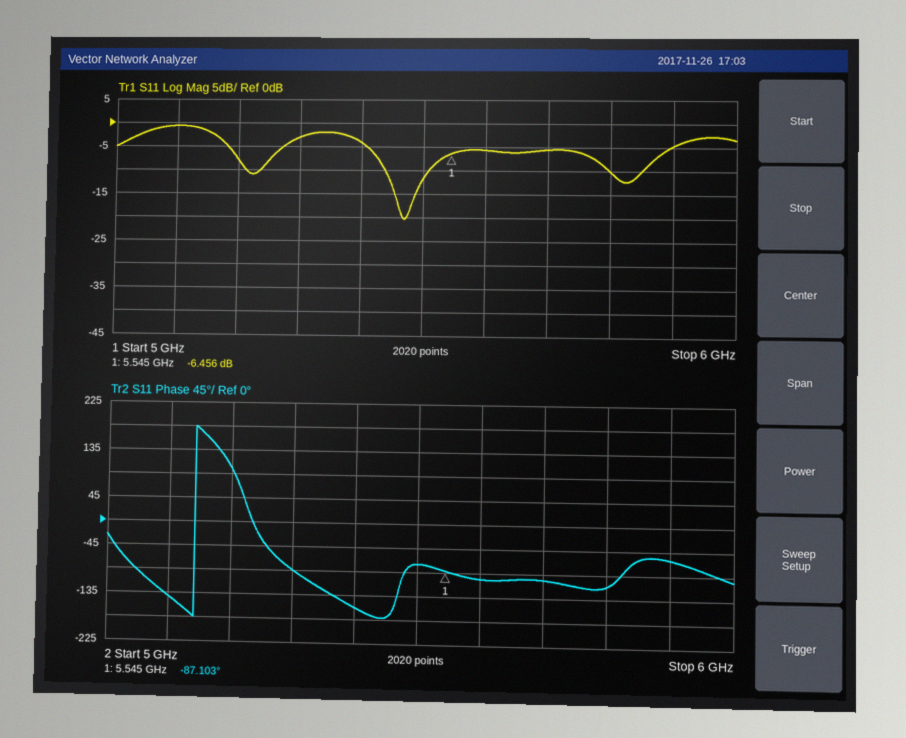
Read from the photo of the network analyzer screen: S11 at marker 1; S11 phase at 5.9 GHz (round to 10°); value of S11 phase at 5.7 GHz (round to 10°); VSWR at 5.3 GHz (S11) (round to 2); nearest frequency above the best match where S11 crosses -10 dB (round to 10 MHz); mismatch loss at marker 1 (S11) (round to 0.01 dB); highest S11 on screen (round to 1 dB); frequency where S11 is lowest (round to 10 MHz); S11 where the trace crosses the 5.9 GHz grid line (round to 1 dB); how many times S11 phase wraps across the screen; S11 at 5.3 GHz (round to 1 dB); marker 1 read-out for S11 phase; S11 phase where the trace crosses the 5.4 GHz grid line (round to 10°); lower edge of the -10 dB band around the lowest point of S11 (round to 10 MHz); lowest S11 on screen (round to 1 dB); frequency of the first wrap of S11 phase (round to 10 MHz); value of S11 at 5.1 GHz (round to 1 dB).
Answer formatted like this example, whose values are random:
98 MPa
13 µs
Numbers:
-6.456 dB
-60°
-100°
6
5.51 GHz
1.11 dB
-1 dB
5.47 GHz
-5 dB
1
-3 dB
-87.103°
-160°
5.44 GHz
-20 dB
5.14 GHz
-1 dB
